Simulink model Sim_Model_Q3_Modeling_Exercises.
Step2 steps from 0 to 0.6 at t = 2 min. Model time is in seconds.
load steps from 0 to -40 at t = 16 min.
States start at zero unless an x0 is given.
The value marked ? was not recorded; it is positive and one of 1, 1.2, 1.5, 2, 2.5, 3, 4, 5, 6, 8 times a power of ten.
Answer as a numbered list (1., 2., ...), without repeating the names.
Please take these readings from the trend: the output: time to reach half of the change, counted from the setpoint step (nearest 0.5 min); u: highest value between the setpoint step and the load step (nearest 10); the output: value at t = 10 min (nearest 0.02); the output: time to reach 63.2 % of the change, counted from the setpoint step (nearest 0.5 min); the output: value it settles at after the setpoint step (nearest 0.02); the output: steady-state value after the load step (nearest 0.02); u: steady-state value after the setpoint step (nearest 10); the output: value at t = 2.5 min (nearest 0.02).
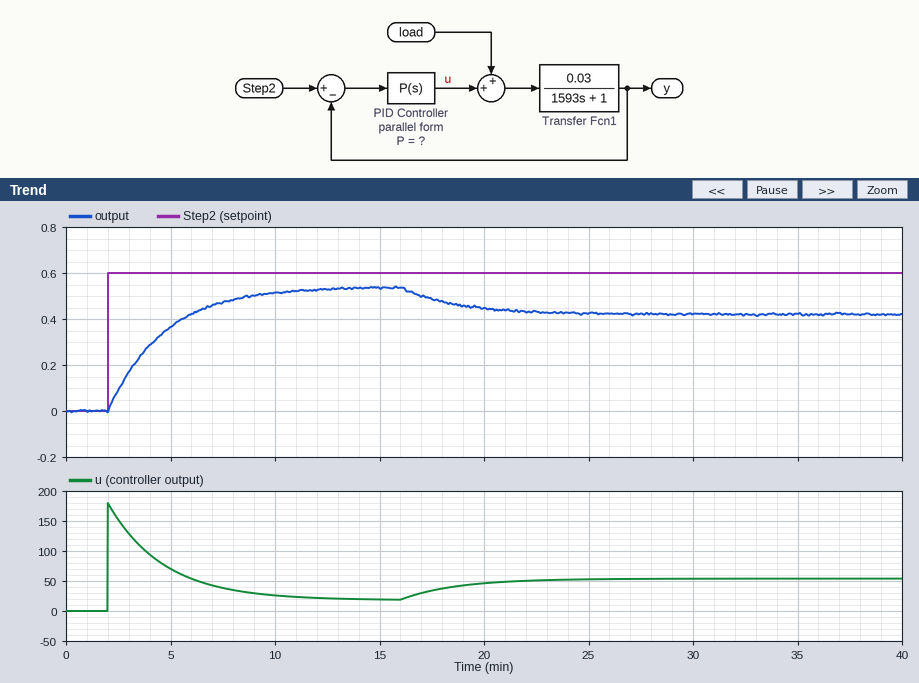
1. 2.0 min
2. 180
3. 0.52
4. 2.5 min
5. 0.54
6. 0.42
7. 20
8. 0.10
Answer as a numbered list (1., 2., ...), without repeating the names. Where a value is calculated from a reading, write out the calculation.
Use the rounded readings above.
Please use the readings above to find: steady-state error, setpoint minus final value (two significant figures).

1. 0.6 - 0.54 = 0.060
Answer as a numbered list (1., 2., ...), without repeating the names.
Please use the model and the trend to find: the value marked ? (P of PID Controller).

1. 300
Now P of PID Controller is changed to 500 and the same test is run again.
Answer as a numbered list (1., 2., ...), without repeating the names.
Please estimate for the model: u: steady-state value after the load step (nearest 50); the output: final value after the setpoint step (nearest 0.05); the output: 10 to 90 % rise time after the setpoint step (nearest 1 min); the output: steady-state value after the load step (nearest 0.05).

1. 50
2. 0.55
3. 4 min
4. 0.50
